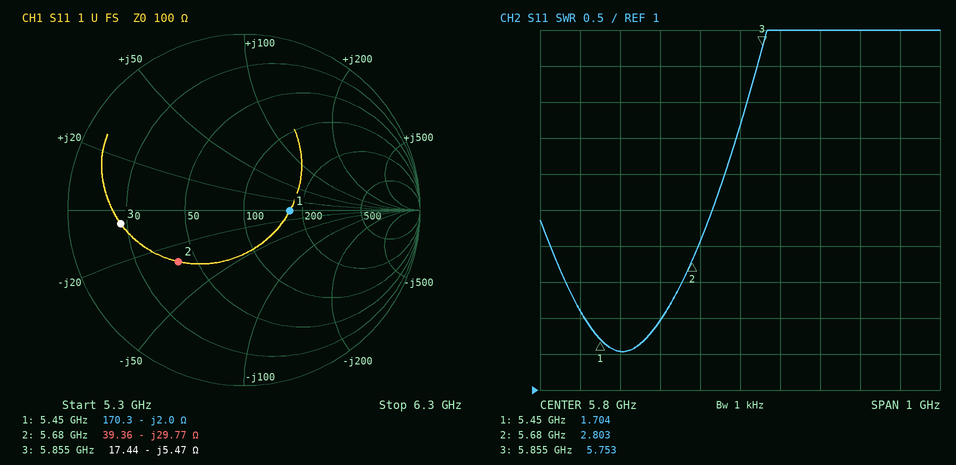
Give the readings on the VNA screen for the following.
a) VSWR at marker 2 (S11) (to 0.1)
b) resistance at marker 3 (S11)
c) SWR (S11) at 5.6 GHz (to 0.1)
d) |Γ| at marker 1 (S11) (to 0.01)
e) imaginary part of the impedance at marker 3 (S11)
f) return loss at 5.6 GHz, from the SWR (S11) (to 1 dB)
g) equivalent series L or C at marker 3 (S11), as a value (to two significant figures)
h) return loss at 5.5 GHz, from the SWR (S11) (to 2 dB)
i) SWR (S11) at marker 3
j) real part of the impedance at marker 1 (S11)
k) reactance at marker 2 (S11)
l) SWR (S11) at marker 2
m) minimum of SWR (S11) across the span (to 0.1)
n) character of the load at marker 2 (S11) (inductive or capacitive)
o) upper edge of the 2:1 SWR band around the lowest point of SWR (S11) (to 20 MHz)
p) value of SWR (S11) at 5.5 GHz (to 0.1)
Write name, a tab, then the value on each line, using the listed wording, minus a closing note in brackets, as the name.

VSWR at marker 2 (S11)	2.8
resistance at marker 3	17.44 Ω
SWR (S11) at 5.6 GHz	2.0
|Γ| at marker 1 (S11)	0.26
imaginary part of the impedance at marker 3	-5.47 Ω
return loss at 5.6 GHz, from the SWR (S11)	10 dB
equivalent series L or C at marker 3 (S11), as a value	5.0 pF
return loss at 5.5 GHz, from the SWR (S11)	14 dB
SWR (S11) at marker 3	5.753
real part of the impedance at marker 1	170.3 Ω
reactance at marker 2	-29.77 Ω
SWR (S11) at marker 2	2.803
minimum of SWR (S11) across the span	1.5
character of the load at marker 2 (S11)	capacitive
upper edge of the 2:1 SWR band around the lowest point of SWR (S11)	5.60 GHz
value of SWR (S11) at 5.5 GHz	1.5
